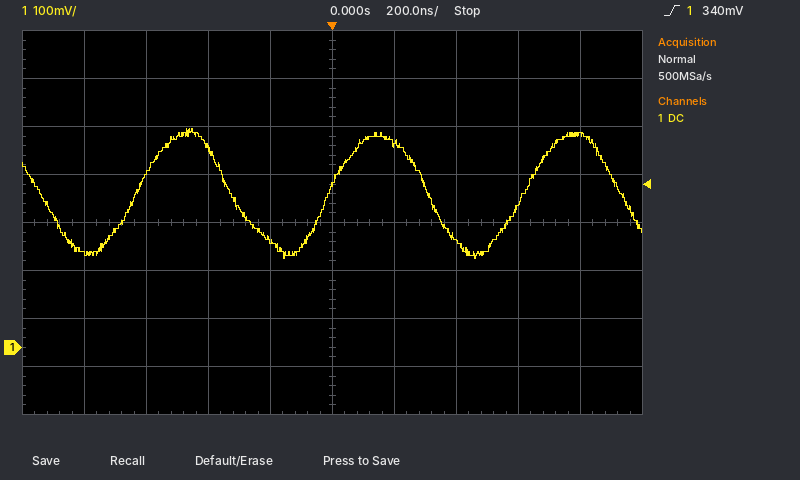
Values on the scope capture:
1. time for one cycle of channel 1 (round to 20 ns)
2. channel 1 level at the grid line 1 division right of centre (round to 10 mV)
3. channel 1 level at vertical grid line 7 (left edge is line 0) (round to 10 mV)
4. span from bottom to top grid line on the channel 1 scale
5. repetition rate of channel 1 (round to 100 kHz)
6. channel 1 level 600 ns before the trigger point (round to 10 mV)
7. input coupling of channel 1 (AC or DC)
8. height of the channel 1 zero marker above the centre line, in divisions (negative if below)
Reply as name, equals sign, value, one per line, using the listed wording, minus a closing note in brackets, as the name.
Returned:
time for one cycle of channel 1 = 620 ns
channel 1 level at the grid line 1 division right of centre = 420 mV
channel 1 level at vertical grid line 7 (left edge is line 0) = 220 mV
span from bottom to top grid line on the channel 1 scale = 800 mV
repetition rate of channel 1 = 1.6 MHz
channel 1 level 600 ns before the trigger point = 360 mV
input coupling of channel 1 = DC
height of the channel 1 zero marker above the centre line, in divisions = -2.6 div
